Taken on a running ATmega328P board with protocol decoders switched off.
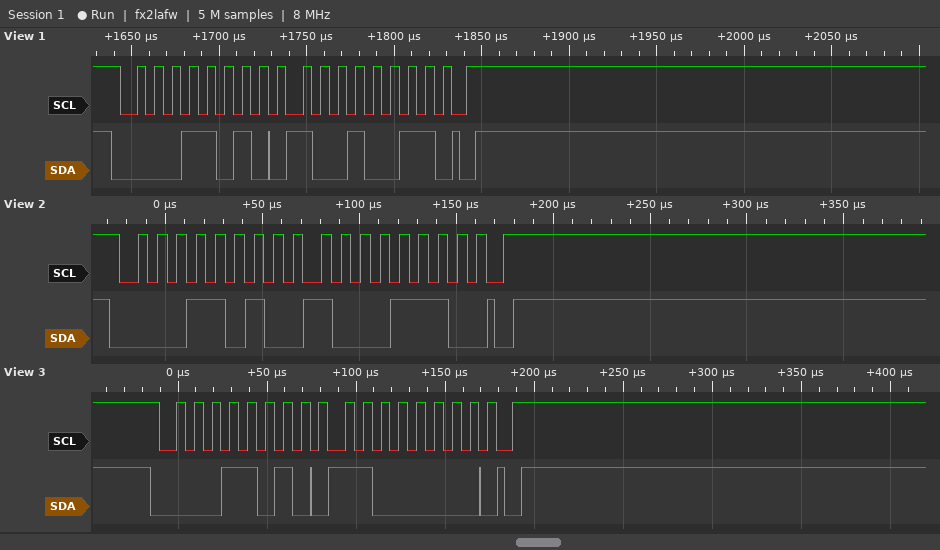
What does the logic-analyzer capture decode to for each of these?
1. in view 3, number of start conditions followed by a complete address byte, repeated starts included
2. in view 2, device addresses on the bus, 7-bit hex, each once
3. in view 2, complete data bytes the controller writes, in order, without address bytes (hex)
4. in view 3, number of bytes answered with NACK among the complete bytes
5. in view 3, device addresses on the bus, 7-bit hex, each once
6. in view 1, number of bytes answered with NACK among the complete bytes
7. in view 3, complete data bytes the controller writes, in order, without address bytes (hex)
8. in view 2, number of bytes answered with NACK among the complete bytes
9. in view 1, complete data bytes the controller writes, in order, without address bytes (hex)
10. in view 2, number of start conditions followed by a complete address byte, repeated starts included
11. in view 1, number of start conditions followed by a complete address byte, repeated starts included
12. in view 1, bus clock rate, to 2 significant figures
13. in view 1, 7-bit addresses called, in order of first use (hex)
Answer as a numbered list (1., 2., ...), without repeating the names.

1. 1
2. 0x0D
3. 8E
4. 0
5. 0x0D
6. 0
7. C0
8. 0
9. 93
10. 1
11. 1
12. 100 kHz
13. 0x0D
